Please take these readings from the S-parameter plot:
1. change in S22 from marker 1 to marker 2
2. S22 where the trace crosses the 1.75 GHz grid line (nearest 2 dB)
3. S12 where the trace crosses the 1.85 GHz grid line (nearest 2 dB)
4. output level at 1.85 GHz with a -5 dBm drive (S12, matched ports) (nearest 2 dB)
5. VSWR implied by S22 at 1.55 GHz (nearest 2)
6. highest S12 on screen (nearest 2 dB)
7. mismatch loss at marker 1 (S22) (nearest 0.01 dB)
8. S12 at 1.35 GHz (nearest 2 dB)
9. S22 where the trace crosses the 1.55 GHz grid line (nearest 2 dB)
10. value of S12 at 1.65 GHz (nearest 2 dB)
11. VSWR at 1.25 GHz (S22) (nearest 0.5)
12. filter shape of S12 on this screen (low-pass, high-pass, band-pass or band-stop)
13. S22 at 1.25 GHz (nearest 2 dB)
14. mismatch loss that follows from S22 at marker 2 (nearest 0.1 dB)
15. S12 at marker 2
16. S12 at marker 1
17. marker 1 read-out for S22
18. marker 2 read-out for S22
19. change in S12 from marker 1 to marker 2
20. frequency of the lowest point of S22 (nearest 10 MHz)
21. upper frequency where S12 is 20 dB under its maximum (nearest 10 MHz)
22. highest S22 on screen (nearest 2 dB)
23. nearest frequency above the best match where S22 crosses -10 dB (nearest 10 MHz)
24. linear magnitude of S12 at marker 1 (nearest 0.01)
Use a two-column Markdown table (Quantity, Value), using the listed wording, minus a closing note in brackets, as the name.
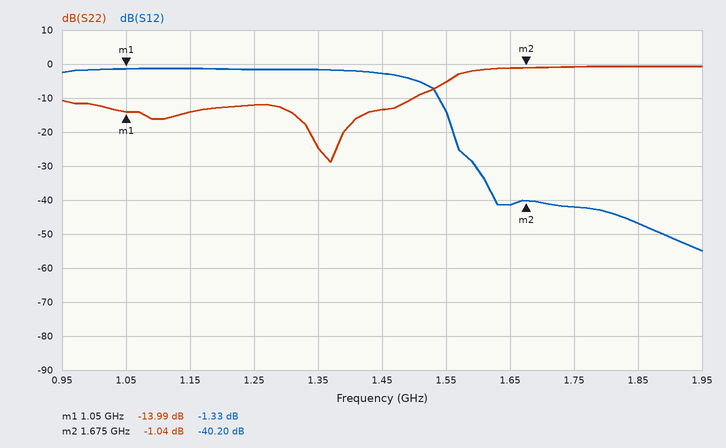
| Quantity | Value |
|---|---|
| change in S22 from marker 1 to marker 2 | 12.95 dB |
| S22 where the trace crosses the 1.75 GHz grid line | 0 dB |
| S12 where the trace crosses the 1.85 GHz grid line | -46 dB |
| output level at 1.85 GHz with a -5 dBm drive (S12, matched ports) | -52 dBm |
| VSWR implied by S22 at 1.55 GHz | 4 |
| highest S12 on screen | -2 dB |
| mismatch loss at marker 1 (S22) | 0.18 dB |
| S12 at 1.35 GHz | -2 dB |
| S22 where the trace crosses the 1.55 GHz grid line | -6 dB |
| value of S12 at 1.65 GHz | -42 dB |
| VSWR at 1.25 GHz (S22) | 1.5 |
| filter shape of S12 on this screen | low-pass |
| S22 at 1.25 GHz | -12 dB |
| mismatch loss that follows from S22 at marker 2 | 6.7 dB |
| S12 at marker 2 | -40.20 dB |
| S12 at marker 1 | -1.33 dB |
| marker 1 read-out for S22 | -13.99 dB |
| marker 2 read-out for S22 | -1.04 dB |
| change in S12 from marker 1 to marker 2 | -38.87 dB |
| frequency of the lowest point of S22 | 1.37 GHz |
| upper frequency where S12 is 20 dB under its maximum | 1.56 GHz |
| highest S22 on screen | 0 dB |
| nearest frequency above the best match where S22 crosses -10 dB | 1.50 GHz |
| linear magnitude of S12 at marker 1 | 0.86 |
